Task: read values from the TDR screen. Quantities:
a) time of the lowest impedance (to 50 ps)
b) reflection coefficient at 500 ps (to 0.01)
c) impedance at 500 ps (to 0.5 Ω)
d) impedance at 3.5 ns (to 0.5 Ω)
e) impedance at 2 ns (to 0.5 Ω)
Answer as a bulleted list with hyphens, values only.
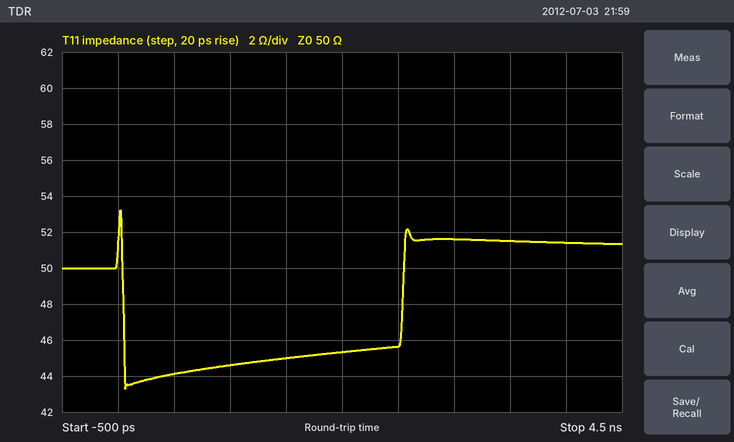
- 50 ps
- -0.06
- 44.0 Ω
- 51.5 Ω
- 45.5 Ω
